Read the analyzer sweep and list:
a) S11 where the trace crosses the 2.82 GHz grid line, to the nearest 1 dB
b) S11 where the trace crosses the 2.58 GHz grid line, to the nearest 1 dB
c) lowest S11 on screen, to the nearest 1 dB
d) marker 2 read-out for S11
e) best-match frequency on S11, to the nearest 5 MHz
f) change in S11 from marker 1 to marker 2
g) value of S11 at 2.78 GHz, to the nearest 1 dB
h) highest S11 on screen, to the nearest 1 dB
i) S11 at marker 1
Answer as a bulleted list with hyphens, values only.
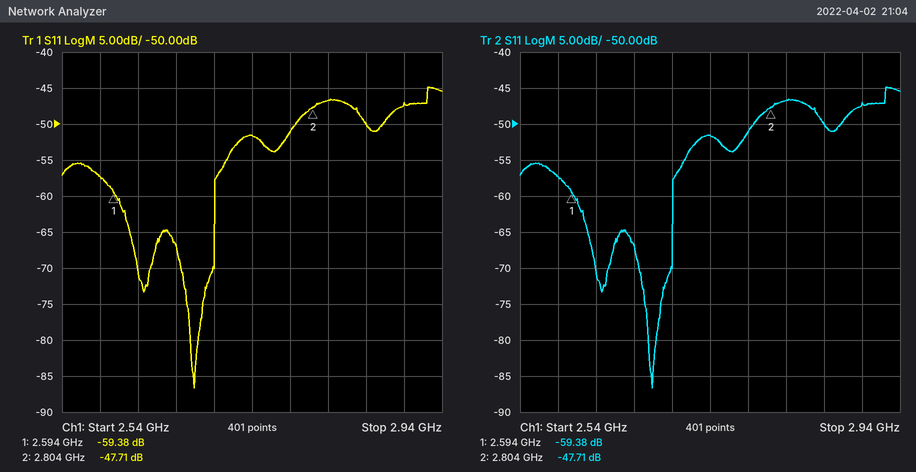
- -47 dB
- -57 dB
- -87 dB
- -47.71 dB
- 2.680 GHz
- 11.67 dB
- -51 dB
- -45 dB
- -59.38 dB
